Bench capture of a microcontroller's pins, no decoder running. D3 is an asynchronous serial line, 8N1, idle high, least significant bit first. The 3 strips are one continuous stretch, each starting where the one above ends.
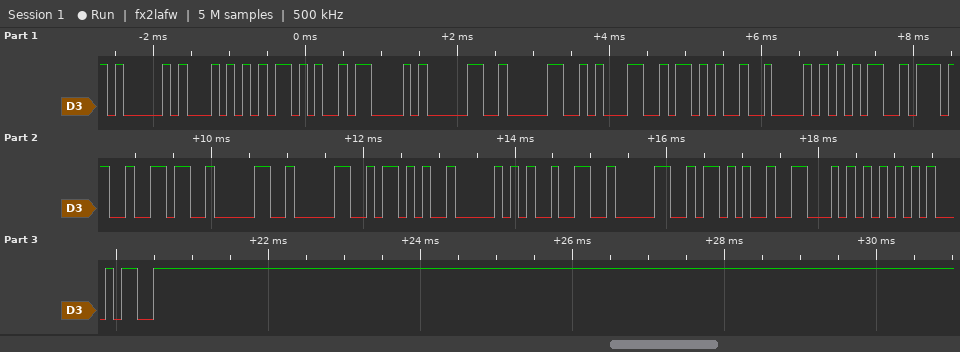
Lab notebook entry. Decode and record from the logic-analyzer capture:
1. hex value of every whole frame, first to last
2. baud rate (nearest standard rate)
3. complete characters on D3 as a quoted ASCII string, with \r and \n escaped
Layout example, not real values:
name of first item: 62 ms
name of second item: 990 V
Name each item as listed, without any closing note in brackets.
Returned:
hex value of every whole frame, first to last: 41 54 2B 43 30 30 31 2B 42 35 37 36 30 30 2B 50 32 30 2B 46 55 34
baud rate: 9600 baud
complete characters on D3 as a quoted ASCII string, with \r and \n escaped: "AT+C001+B57600+P20+FU4"
